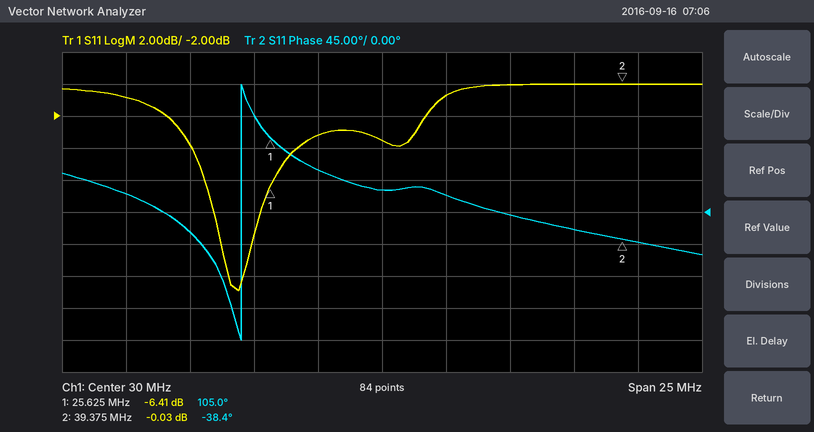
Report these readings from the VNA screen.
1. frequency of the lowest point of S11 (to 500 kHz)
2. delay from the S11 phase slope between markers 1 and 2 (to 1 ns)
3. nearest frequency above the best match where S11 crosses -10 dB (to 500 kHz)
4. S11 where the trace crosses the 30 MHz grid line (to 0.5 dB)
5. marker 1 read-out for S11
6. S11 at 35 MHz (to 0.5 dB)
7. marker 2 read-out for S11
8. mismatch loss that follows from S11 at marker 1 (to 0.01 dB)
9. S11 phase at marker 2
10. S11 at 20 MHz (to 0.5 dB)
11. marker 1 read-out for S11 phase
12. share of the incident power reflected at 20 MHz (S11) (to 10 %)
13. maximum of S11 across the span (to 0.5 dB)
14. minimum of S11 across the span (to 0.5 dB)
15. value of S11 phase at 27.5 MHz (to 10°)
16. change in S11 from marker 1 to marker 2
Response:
24.5 MHz
29 ns
25.0 MHz
-3.5 dB
-6.41 dB
0.0 dB
-0.03 dB
1.13 dB
-38.4°
-1.0 dB
105.0°
80 %
0.0 dB
-13.0 dB
60°
6.38 dB
